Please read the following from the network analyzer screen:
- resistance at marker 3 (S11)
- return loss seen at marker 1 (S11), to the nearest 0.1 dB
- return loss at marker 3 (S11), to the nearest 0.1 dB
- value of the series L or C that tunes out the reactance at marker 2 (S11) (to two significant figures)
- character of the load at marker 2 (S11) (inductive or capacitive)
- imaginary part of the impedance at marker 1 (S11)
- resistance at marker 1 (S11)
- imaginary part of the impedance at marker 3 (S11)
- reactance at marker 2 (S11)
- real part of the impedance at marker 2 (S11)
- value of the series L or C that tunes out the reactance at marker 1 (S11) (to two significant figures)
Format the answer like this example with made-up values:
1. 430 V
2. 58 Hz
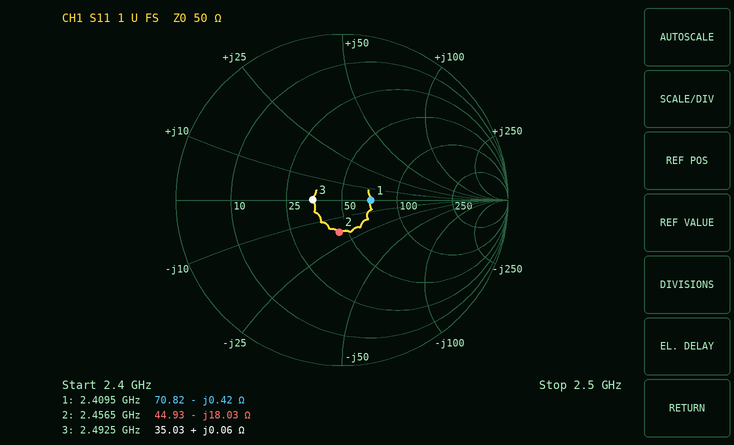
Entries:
1. 35.03 Ω
2. 15.3 dB
3. 15.1 dB
4. 1.2 nH
5. capacitive
6. -0.42 Ω
7. 70.82 Ω
8. +0.06 Ω
9. -18.03 Ω
10. 44.93 Ω
11. 28 pH
